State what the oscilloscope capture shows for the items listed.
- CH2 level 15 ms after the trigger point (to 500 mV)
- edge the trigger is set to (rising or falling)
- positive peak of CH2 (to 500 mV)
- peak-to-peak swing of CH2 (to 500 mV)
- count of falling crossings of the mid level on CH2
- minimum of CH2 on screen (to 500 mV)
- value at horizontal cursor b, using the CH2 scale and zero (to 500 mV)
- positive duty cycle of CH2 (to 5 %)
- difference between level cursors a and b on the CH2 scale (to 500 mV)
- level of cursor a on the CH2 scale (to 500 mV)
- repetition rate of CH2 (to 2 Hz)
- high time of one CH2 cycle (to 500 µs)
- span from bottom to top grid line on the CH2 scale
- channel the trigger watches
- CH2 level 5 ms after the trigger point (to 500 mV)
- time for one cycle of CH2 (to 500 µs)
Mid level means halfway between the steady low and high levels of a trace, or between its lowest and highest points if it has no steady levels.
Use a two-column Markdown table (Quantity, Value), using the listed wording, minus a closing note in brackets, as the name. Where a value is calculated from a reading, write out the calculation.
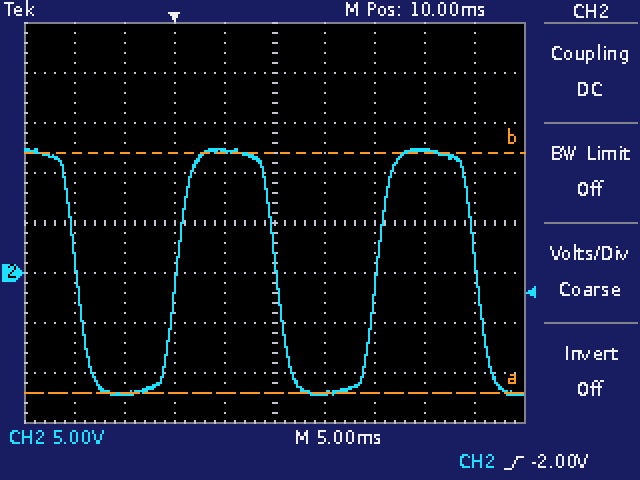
| Quantity | Value |
|---|---|
| CH2 level 15 ms after the trigger point | -12.0 V |
| edge the trigger is set to | rising |
| positive peak of CH2 | 12.5 V |
| peak-to-peak swing of CH2 | 12.5 V − (-12.0 V) = 24.5 V |
| count of falling crossings of the mid level on CH2 | 3 |
| minimum of CH2 on screen | -12.0 V |
| value at horizontal cursor b, using the CH2 scale and zero | 12.0 V |
| positive duty cycle of CH2 | 10.0 ms / 20.0 ms ≈ 50 % |
| difference between level cursors a and b on the CH2 scale | 24.0 V |
| level of cursor a on the CH2 scale | -12.0 V |
| repetition rate of CH2 | 1 / 20.0 ms ≈ 50 Hz |
| high time of one CH2 cycle | 10.0 ms |
| span from bottom to top grid line on the CH2 scale | 40 V |
| channel the trigger watches | CH2 |
| CH2 level 5 ms after the trigger point | 12.0 V |
| time for one cycle of CH2 | 20.0 ms |
